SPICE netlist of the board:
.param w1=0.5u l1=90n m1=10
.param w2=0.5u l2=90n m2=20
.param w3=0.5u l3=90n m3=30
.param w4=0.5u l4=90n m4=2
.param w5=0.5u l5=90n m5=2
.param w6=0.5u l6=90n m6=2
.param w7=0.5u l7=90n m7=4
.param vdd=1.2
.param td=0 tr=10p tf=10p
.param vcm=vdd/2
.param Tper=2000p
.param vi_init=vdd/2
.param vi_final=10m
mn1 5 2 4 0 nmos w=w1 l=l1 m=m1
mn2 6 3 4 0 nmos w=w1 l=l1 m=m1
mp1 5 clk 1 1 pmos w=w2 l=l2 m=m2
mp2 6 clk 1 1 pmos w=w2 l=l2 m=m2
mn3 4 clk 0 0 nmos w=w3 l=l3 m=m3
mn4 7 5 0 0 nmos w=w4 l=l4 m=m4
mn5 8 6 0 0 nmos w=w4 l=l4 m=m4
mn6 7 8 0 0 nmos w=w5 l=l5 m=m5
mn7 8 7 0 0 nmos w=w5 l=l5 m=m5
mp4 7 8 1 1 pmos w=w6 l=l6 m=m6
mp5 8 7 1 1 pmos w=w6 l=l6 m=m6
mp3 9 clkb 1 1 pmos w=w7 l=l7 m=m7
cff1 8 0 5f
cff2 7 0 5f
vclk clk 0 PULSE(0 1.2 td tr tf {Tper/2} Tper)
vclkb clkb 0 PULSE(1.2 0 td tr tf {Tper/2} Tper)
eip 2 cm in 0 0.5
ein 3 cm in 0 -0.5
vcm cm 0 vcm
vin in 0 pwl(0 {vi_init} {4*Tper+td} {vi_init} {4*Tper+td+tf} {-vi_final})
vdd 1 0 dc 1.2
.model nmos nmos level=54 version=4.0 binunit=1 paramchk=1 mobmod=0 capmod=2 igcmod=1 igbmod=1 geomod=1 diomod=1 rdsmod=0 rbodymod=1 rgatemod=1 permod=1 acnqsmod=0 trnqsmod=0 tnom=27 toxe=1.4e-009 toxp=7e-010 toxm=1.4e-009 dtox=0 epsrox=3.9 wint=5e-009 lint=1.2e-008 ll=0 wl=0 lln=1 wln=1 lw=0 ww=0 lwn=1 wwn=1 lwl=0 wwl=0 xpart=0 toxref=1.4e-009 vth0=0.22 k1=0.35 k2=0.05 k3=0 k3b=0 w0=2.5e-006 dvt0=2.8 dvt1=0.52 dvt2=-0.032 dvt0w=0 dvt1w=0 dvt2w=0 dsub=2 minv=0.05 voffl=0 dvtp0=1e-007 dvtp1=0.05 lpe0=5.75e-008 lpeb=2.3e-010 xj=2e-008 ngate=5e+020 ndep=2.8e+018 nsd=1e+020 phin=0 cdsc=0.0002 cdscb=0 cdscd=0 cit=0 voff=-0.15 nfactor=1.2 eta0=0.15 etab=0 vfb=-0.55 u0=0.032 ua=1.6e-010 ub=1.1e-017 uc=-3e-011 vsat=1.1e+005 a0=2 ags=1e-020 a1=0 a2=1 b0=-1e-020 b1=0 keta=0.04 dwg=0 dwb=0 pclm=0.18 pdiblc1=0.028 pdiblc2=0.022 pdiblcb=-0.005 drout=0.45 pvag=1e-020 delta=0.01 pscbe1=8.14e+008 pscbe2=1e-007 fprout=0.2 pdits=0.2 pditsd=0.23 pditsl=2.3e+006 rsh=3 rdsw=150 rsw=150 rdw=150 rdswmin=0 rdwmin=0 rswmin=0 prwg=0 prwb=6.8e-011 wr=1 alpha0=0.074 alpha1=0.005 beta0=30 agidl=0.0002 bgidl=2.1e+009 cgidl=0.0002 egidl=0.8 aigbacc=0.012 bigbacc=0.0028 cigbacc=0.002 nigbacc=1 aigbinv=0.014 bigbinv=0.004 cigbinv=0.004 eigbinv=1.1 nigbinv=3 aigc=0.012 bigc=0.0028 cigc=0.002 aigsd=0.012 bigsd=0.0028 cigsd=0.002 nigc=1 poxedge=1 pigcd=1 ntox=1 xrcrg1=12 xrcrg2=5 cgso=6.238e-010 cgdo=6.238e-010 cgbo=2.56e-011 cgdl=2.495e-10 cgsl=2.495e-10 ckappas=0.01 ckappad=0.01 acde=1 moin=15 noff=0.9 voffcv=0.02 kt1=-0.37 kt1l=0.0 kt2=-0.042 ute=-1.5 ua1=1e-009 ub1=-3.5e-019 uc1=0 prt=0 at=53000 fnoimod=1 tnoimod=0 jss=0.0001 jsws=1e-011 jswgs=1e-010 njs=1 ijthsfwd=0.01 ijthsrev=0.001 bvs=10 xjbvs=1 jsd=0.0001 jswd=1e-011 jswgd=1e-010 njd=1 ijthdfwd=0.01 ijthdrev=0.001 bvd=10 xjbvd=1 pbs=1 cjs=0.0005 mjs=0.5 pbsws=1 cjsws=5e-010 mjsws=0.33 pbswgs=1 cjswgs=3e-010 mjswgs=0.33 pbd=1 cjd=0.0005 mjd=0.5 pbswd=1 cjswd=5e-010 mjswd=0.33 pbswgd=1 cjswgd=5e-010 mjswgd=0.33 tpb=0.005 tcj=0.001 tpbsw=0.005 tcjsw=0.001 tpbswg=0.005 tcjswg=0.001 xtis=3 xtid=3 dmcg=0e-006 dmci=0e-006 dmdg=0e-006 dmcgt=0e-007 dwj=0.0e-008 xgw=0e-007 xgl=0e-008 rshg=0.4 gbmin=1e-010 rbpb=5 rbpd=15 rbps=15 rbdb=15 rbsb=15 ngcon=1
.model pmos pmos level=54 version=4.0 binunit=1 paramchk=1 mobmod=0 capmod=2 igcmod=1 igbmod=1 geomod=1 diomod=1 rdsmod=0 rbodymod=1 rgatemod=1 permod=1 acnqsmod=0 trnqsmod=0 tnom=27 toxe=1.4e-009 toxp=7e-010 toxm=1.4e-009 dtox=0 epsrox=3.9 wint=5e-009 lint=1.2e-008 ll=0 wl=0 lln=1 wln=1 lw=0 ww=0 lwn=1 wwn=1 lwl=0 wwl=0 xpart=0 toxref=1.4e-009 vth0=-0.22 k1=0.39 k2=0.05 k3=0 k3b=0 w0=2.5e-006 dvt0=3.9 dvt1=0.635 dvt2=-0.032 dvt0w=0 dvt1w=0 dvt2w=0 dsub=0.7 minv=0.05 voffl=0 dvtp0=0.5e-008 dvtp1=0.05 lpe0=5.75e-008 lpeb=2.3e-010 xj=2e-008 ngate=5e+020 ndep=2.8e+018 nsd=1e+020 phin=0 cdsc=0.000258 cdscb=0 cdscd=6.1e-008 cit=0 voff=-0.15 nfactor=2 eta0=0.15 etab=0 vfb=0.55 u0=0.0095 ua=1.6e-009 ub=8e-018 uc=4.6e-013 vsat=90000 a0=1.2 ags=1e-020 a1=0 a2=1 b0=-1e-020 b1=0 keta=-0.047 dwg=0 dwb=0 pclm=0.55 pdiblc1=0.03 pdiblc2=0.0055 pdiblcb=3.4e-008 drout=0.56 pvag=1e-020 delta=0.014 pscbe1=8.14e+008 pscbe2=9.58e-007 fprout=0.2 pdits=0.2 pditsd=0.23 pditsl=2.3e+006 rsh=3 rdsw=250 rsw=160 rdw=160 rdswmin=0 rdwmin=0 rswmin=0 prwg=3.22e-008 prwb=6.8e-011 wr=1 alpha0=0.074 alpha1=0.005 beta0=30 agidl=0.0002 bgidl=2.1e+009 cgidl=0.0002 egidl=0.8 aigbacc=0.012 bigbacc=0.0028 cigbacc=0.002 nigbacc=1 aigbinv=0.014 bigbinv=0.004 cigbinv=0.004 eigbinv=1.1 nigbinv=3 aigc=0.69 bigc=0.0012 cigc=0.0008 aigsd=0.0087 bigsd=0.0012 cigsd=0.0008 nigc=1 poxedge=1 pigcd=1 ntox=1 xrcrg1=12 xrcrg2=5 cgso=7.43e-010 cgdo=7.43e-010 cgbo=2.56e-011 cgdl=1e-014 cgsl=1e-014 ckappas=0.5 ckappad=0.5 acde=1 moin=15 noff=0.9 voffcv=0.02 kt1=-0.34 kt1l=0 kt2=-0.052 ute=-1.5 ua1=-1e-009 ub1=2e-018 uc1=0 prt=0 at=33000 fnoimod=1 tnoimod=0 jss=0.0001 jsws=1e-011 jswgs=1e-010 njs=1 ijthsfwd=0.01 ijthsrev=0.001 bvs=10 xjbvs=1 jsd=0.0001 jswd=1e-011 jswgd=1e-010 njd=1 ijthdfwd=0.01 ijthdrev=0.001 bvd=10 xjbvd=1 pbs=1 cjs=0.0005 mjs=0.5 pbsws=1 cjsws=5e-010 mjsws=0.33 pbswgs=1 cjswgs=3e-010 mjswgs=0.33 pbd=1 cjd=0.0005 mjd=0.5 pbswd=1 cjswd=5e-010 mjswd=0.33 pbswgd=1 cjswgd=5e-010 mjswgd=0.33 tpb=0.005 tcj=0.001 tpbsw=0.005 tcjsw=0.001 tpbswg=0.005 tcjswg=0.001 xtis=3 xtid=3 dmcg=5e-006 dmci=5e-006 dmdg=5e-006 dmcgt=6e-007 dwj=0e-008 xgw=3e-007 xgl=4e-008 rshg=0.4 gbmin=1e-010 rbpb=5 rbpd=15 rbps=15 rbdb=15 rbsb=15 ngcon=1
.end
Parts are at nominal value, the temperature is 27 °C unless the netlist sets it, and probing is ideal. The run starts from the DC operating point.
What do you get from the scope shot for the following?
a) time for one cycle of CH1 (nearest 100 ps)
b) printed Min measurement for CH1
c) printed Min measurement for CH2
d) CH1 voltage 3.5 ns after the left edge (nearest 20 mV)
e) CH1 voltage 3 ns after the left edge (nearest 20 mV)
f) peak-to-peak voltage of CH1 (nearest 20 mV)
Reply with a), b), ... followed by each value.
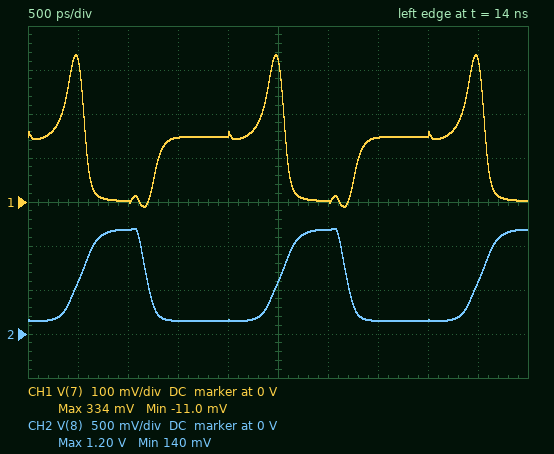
a) 2.0 ns
b) -11.0 mV
c) 140 mV
d) 140 mV
e) 0 V
f) 340 mV
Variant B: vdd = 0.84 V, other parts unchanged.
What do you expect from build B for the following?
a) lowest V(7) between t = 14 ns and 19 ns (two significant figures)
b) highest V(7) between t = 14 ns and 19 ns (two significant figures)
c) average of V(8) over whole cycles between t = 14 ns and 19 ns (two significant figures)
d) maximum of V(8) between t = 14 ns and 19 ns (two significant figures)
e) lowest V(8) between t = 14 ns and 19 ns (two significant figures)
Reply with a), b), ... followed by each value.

a) -9.4 mV
b) 280 mV
c) 360 mV
d) 840 mV
e) 77 mV
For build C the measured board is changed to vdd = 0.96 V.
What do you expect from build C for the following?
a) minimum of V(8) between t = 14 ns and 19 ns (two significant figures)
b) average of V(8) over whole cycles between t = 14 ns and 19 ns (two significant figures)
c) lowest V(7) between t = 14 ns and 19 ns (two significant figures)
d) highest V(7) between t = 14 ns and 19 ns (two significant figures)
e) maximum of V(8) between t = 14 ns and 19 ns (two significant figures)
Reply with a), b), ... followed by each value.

a) 98 mV
b) 410 mV
c) -10 mV
d) 310 mV
e) 960 mV
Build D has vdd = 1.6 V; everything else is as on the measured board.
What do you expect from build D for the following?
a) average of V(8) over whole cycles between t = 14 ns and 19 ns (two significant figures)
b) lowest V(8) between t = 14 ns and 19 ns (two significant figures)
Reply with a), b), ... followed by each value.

a) 560 mV
b) 220 mV
